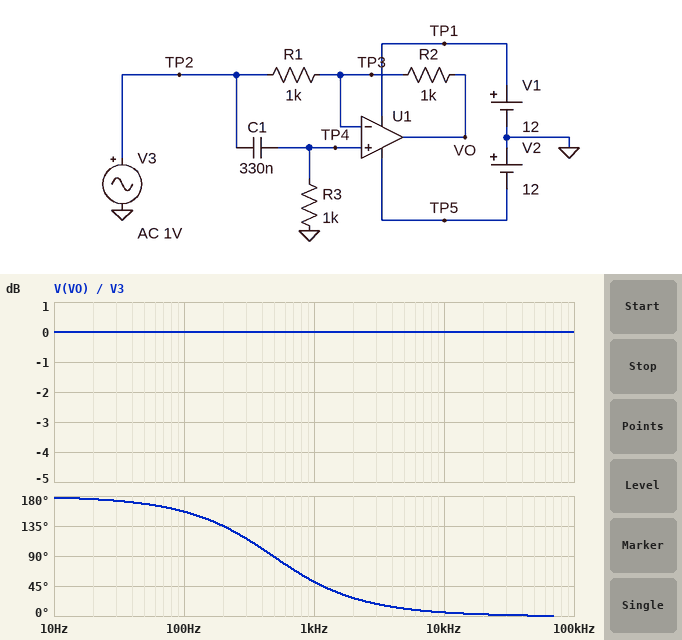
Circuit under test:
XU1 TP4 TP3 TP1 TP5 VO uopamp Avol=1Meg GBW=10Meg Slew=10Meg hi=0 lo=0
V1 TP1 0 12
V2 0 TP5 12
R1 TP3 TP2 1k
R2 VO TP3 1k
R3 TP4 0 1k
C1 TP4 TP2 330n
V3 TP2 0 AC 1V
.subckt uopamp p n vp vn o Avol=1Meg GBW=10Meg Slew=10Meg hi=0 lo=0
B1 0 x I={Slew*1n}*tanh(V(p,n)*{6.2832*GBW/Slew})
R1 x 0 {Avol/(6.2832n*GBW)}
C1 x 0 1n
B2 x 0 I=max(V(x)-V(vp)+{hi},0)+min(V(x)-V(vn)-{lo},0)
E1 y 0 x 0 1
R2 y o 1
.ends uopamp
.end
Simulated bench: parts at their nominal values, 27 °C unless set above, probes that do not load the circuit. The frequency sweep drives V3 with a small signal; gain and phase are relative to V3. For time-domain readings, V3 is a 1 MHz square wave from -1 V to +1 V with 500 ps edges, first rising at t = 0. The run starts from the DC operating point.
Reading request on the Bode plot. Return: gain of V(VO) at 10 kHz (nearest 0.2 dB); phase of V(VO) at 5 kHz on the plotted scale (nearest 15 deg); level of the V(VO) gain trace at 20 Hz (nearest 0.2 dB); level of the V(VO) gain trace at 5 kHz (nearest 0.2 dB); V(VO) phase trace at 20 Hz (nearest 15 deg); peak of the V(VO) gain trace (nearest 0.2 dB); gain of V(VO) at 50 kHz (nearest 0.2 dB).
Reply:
0 dB
15 deg
0 dB
0 dB
180 deg
0 dB
0 dB
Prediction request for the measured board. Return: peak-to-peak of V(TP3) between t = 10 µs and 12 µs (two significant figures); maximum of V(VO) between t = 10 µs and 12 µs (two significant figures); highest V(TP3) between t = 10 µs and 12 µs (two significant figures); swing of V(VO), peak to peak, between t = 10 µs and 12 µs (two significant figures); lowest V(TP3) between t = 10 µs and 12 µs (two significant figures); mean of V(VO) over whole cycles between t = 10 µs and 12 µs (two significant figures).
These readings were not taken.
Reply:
2.0 V
2.9 V
2.0 V
2.0 V
-36 mV
1.9 V
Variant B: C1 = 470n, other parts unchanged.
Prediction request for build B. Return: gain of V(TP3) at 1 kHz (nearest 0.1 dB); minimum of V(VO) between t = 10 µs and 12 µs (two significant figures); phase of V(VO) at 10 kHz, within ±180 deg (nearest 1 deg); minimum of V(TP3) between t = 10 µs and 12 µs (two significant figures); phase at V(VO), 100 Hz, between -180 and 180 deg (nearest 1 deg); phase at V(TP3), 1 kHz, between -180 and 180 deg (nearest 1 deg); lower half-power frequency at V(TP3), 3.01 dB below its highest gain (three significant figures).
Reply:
-0.5 dB
950 mV
4 deg
-25 mV
147 deg
19 deg
339 Hz
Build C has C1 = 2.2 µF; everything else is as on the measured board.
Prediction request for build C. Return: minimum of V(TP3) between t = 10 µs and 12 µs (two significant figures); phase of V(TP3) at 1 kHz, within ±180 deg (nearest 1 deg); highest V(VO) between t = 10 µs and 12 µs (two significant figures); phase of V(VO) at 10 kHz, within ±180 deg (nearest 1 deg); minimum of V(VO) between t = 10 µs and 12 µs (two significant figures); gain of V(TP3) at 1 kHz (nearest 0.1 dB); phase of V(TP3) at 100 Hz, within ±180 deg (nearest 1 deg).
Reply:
-5.4 mV
4 deg
3.0 V
1 deg
990 mV
0 dB
36 deg
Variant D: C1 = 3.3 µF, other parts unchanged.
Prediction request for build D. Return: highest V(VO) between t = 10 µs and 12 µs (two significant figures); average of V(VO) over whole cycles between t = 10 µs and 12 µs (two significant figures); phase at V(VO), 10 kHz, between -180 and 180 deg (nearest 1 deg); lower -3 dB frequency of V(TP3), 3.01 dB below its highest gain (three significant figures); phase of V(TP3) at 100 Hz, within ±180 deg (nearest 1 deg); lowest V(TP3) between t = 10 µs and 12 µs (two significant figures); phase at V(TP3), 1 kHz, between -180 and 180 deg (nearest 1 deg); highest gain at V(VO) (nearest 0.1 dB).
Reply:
3.0 V
2.0 V
0 deg
48.2 Hz
26 deg
-3.6 mV
3 deg
0 dB
